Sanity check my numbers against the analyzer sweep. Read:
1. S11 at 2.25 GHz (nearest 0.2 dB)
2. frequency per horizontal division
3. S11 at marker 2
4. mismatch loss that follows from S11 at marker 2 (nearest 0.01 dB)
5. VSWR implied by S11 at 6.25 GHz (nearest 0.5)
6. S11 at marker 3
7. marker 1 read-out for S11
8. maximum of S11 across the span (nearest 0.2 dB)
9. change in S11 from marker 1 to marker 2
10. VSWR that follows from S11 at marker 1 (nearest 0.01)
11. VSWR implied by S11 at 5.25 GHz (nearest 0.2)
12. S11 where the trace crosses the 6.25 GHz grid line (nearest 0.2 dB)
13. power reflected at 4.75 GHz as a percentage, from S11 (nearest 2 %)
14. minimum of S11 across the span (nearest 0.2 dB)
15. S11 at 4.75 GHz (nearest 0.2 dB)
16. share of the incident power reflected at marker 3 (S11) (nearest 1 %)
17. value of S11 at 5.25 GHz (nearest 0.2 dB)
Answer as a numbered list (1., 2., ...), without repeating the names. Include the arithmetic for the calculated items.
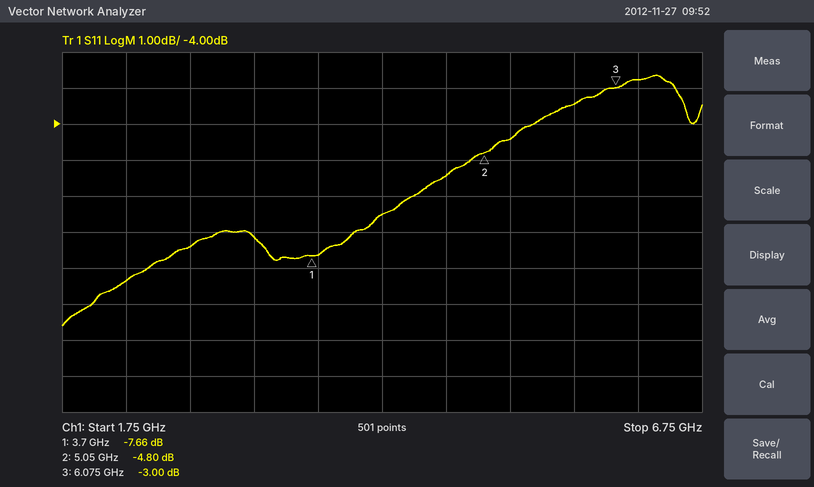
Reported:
1. -8.4 dB
2. 500 MHz
3. -4.80 dB
4. −10 log10(1 − 10^(-4.8/10)) ≈ 1.75 dB
5. |Γ| = 10^(-2.8/20) = 0.7244; VSWR = (1 + 0.7244)/(1 − 0.7244) ≈ 6.26, so 6.5 to the nearest 0.5
6. -3.00 dB
7. -7.66 dB
8. -2.6 dB
9. -4.8 − (-7.66) = 2.86 dB
10. (1 + 0.4140)/(1 − 0.4140) ≈ 2.41
11. |Γ| = 10^(-4.4/20) = 0.6026; VSWR = (1 + 0.6026)/(1 − 0.6026) ≈ 4.0
12. -2.8 dB
13. 10^(-5.4/10) ≈ 28.8 %, so 28 % to the nearest 2 %
14. -9.6 dB
15. -5.4 dB
16. 10^(-3/10) ≈ 50 %
17. -4.4 dB
